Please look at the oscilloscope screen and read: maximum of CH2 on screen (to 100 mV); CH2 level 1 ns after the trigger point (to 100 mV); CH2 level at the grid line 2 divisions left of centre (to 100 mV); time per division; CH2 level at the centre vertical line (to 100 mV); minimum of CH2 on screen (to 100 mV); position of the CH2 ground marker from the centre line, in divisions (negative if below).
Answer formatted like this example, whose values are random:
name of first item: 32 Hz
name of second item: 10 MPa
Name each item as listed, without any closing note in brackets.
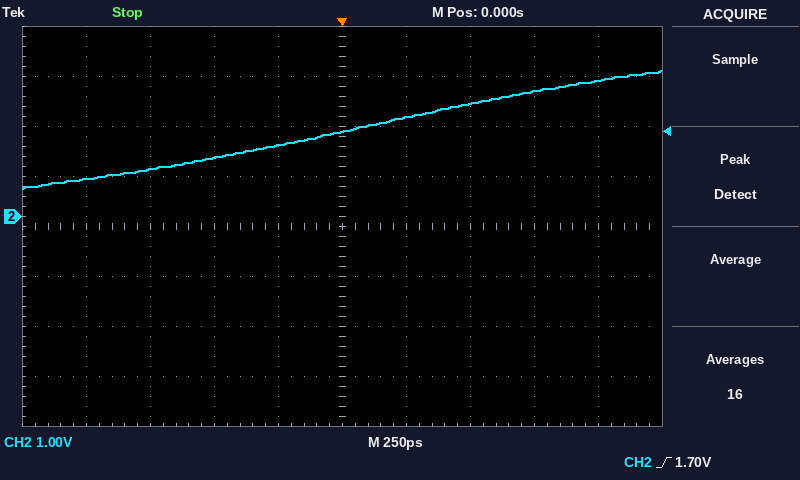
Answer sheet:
maximum of CH2 on screen: 2.9 V
CH2 level 1 ns after the trigger point: 2.7 V
CH2 level at the grid line 2 divisions left of centre: 1.2 V
time per division: 250 ps
CH2 level at the centre vertical line: 1.7 V
minimum of CH2 on screen: 600 mV
position of the CH2 ground marker from the centre line, in divisions: +0.2 div
